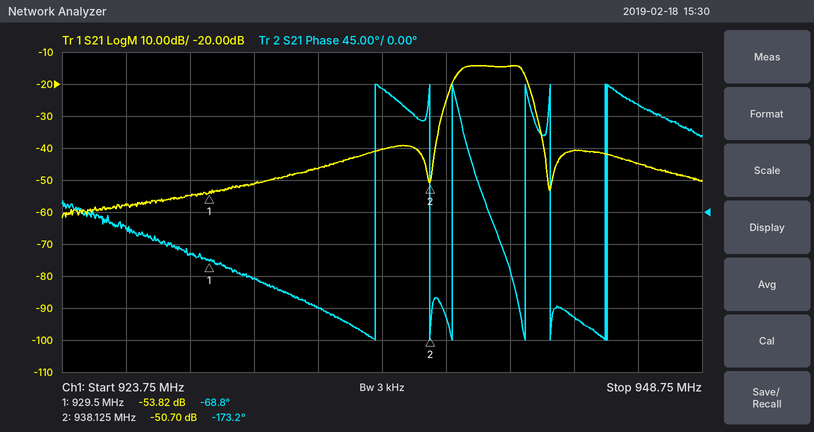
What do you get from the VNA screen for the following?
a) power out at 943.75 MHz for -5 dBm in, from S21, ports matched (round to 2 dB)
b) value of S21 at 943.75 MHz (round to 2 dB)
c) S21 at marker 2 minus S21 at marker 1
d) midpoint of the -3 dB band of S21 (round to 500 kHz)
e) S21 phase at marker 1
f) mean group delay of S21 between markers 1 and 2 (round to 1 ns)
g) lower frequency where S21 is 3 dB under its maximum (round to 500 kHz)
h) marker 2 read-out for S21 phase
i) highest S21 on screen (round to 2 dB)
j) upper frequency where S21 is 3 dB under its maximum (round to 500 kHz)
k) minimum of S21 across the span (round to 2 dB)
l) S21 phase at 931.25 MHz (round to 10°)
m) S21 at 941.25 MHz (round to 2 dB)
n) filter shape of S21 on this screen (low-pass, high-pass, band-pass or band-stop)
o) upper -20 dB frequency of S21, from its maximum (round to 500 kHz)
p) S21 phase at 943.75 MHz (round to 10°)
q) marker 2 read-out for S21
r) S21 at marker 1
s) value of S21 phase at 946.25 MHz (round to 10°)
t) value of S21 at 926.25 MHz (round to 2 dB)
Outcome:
-46 dBm
-40 dB
3.12 dB
940.5 MHz
-68.8°
34 ns
939.0 MHz
-173.2°
-14 dB
942.0 MHz
-62 dB
-90°
-14 dB
band-pass
942.5 MHz
-150°
-50.70 dB
-53.82 dB
150°
-58 dB
